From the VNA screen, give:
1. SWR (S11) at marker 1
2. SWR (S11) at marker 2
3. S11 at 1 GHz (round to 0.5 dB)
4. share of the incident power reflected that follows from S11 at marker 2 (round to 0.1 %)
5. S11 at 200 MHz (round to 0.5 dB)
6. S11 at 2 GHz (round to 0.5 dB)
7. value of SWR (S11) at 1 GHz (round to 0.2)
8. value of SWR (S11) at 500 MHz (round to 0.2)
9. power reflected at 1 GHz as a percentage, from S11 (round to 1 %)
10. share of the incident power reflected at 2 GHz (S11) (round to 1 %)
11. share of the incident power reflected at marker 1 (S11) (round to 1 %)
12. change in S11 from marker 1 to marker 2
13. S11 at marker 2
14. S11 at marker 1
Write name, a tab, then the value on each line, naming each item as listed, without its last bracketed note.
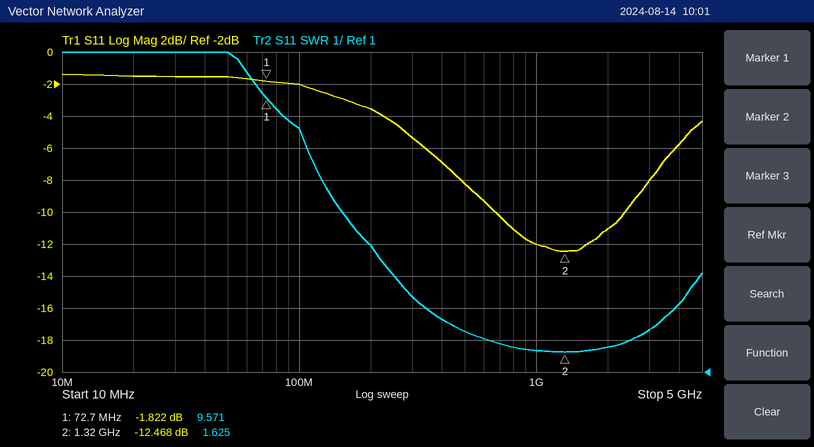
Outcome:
SWR (S11) at marker 1	9.571
SWR (S11) at marker 2	1.625
S11 at 1 GHz	-12.0 dB
share of the incident power reflected that follows from S11 at marker 2	5.7 %
S11 at 200 MHz	-3.5 dB
S11 at 2 GHz	-11.0 dB
value of SWR (S11) at 1 GHz	1.6
value of SWR (S11) at 500 MHz	2.2
power reflected at 1 GHz as a percentage, from S11	6 %
share of the incident power reflected at 2 GHz (S11)	8 %
share of the incident power reflected at marker 1 (S11)	66 %
change in S11 from marker 1 to marker 2	-10.646 dB
S11 at marker 2	-12.468 dB
S11 at marker 1	-1.822 dB
